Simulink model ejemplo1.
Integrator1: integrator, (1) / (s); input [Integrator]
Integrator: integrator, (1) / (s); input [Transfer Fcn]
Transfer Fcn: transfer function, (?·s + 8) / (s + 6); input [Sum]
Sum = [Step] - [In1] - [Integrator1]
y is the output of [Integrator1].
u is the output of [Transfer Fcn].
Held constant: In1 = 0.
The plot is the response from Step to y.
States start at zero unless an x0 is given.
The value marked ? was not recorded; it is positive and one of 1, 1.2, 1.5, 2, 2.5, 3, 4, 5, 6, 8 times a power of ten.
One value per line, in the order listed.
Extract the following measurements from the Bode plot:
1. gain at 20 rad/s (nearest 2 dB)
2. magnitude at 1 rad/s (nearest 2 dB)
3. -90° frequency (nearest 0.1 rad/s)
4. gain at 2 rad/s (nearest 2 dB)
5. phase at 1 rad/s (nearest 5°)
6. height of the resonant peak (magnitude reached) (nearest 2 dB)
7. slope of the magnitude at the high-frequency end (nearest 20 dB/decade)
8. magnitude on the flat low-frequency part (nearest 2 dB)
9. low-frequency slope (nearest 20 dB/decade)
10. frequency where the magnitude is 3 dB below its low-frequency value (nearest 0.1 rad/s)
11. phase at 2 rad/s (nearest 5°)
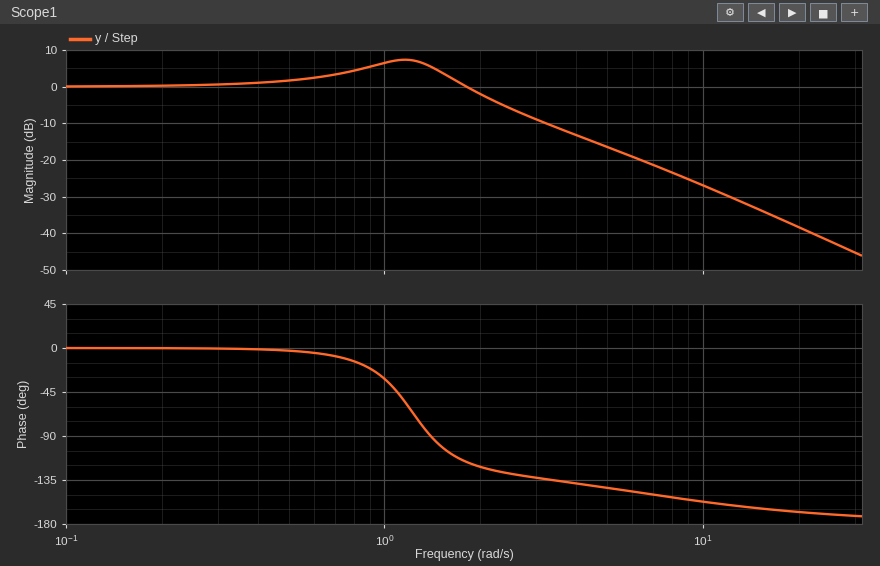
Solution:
-38 dB
6 dB
1.4 rad/s
-2 dB
-30°
8 dB
-40 dB/decade
0 dB
0 dB/decade
2.1 rad/s
-120°
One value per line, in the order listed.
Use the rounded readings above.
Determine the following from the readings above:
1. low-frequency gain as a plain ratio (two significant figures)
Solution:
1.0
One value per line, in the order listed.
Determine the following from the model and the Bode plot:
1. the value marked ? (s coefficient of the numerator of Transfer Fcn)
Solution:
5
